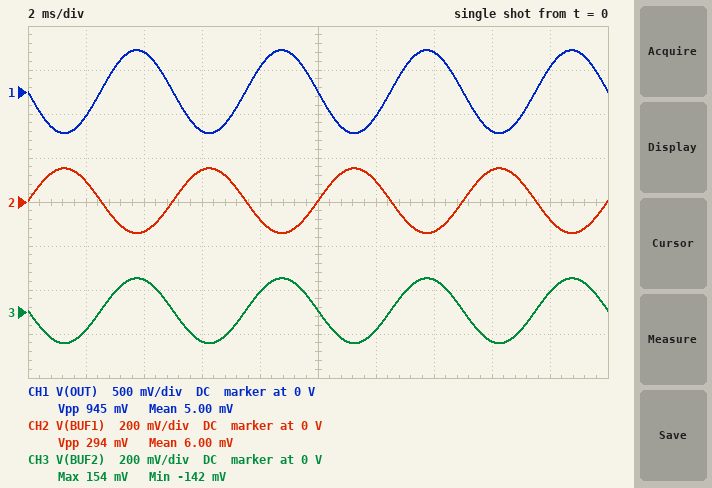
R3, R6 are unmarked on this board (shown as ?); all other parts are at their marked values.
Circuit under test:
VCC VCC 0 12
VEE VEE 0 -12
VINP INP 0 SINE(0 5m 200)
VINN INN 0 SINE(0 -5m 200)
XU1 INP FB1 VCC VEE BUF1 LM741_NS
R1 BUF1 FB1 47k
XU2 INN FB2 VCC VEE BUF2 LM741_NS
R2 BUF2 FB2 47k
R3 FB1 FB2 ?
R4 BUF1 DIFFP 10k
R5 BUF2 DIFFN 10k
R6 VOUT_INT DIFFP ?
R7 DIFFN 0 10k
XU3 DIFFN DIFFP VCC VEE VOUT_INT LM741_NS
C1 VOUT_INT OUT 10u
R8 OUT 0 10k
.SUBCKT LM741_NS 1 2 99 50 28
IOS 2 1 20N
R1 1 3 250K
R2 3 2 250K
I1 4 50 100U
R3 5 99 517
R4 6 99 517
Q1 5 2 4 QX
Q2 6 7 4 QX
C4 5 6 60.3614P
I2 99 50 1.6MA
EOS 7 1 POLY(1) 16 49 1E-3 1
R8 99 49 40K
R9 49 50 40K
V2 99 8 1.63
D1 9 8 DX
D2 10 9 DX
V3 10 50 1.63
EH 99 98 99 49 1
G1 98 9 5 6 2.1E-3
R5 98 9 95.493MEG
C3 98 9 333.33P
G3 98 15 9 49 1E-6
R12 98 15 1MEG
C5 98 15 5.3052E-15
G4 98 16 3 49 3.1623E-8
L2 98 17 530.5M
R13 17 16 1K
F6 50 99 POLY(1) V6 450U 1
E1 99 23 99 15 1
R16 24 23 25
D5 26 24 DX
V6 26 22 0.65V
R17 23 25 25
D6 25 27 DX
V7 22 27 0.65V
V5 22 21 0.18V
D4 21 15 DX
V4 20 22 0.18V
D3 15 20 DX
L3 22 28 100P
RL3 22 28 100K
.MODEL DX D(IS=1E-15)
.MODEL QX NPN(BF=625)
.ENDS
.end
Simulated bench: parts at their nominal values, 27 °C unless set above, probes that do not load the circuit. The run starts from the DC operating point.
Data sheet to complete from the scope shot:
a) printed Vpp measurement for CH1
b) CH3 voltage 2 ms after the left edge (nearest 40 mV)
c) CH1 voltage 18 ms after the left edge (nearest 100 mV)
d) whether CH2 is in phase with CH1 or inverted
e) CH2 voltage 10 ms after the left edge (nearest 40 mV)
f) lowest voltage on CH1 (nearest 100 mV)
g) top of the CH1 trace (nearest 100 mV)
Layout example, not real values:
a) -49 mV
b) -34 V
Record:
a) 945 mV
b) -80 mV
c) 300 mV
d) inverted
e) 0 V
f) -500 mV
g) 500 mV
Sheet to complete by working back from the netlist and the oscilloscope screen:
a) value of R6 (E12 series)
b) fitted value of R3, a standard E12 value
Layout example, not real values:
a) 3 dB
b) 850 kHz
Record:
a) 18 kΩ
b) 3.3 kΩ
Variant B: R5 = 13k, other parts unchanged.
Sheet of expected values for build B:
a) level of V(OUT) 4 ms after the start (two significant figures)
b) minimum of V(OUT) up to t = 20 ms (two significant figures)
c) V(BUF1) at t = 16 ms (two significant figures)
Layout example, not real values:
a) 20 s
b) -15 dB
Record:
a) 430 mV
b) -440 mV
c) 150 mV
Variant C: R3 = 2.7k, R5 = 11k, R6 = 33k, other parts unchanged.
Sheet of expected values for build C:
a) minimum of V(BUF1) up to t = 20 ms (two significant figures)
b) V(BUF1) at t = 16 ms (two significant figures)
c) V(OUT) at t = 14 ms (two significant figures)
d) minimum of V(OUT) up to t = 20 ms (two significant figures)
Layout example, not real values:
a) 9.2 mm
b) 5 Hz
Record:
a) -170 mV
b) 180 mV
c) 920 mV
d) -950 mV
